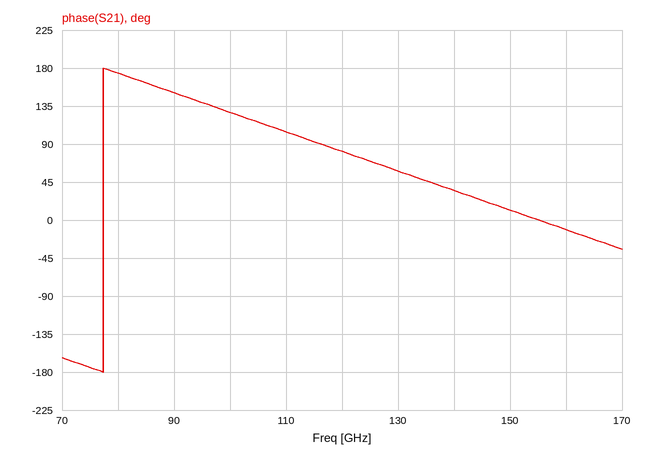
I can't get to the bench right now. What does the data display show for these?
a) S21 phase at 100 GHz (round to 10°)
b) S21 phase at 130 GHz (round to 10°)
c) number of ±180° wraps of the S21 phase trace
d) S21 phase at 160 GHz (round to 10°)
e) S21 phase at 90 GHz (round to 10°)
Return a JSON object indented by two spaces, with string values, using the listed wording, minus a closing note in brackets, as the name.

{
  "S21 phase at 100 GHz": "130°",
  "S21 phase at 130 GHz": "60°",
  "number of ±180° wraps of the S21 phase trace": "1",
  "S21 phase at 160 GHz": "-10°",
  "S21 phase at 90 GHz": "150°"
}
